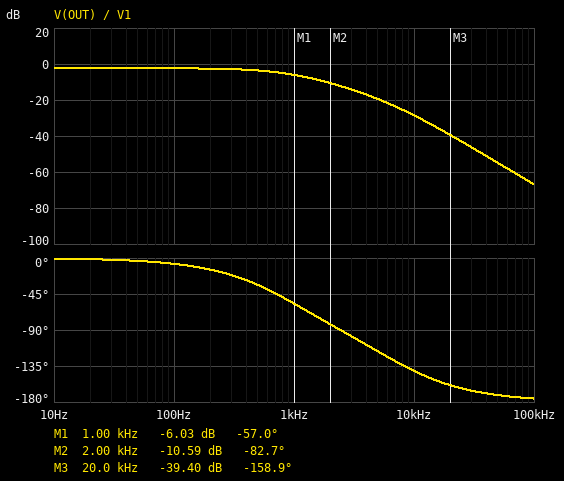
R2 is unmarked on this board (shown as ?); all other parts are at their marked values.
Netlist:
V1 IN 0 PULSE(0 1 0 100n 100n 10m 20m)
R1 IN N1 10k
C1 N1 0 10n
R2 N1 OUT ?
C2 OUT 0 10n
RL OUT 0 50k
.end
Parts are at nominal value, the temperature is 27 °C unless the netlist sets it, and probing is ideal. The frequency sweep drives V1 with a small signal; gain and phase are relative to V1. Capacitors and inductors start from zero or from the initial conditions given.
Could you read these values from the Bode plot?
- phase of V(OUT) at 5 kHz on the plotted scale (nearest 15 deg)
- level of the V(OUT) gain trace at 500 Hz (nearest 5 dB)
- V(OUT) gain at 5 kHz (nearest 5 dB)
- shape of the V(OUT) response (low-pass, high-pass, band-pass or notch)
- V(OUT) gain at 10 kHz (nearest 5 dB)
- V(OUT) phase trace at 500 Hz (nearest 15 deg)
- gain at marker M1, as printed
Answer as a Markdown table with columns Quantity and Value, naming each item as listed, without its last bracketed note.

| Quantity | Value |
|---|---|
| phase of V(OUT) at 5 kHz on the plotted scale | -120 deg |
| level of the V(OUT) gain trace at 500 Hz | -5 dB |
| V(OUT) gain at 5 kHz | -20 dB |
| shape of the V(OUT) response | low-pass |
| V(OUT) gain at 10 kHz | -30 dB |
| V(OUT) phase trace at 500 Hz | -30 deg |
| gain at marker M1, as printed | -6.03 dB |
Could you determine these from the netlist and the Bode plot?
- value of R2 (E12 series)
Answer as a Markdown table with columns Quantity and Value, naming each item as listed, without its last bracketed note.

| Quantity | Value |
|---|---|
| value of R2 | 5.6 kΩ |
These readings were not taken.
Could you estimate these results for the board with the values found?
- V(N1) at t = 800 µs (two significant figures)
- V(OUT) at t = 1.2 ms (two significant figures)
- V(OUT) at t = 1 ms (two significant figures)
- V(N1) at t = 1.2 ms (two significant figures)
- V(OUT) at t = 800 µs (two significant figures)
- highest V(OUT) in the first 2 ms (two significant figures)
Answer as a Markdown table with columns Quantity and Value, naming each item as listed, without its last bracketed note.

| Quantity | Value |
|---|---|
| V(N1) at t = 800 µs | 840 mV |
| V(OUT) at t = 1.2 ms | 760 mV |
| V(OUT) at t = 1 ms | 760 mV |
| V(N1) at t = 1.2 ms | 850 mV |
| V(OUT) at t = 800 µs | 750 mV |
| highest V(OUT) in the first 2 ms | 760 mV |
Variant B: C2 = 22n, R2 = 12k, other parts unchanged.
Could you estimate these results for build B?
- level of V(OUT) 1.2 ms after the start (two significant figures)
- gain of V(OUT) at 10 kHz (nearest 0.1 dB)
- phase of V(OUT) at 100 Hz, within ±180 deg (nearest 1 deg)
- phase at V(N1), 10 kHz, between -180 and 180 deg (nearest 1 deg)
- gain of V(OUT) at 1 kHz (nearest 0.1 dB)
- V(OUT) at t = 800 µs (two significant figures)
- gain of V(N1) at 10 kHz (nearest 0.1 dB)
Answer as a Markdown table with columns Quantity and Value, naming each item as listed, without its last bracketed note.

| Quantity | Value |
|---|---|
| level of V(OUT) 1.2 ms after the start | 660 mV |
| gain of V(OUT) at 10 kHz | -40.8 dB |
| phase of V(OUT) at 100 Hz, within ±180 deg | -15 deg |
| phase at V(N1), 10 kHz, between -180 and 180 deg | -74 deg |
| gain of V(OUT) at 1 kHz | -11.7 dB |
| V(OUT) at t = 800 µs | 600 mV |
| gain of V(N1) at 10 kHz | -16.4 dB |
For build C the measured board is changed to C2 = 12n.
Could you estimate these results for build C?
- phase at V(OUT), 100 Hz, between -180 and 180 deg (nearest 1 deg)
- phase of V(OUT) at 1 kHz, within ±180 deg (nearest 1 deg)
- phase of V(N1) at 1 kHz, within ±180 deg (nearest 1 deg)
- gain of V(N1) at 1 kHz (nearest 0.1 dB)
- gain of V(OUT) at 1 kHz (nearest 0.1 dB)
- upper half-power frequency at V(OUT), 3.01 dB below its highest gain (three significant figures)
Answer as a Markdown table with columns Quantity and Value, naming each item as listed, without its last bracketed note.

| Quantity | Value |
|---|---|
| phase at V(OUT), 100 Hz, between -180 and 180 deg | -8 deg |
| phase of V(OUT) at 1 kHz, within ±180 deg | -61 deg |
| phase of V(N1) at 1 kHz, within ±180 deg | -40 deg |
| gain of V(N1) at 1 kHz | -5.1 dB |
| gain of V(OUT) at 1 kHz | -6.6 dB |
| upper half-power frequency at V(OUT), 3.01 dB below its highest gain | 776 Hz |
